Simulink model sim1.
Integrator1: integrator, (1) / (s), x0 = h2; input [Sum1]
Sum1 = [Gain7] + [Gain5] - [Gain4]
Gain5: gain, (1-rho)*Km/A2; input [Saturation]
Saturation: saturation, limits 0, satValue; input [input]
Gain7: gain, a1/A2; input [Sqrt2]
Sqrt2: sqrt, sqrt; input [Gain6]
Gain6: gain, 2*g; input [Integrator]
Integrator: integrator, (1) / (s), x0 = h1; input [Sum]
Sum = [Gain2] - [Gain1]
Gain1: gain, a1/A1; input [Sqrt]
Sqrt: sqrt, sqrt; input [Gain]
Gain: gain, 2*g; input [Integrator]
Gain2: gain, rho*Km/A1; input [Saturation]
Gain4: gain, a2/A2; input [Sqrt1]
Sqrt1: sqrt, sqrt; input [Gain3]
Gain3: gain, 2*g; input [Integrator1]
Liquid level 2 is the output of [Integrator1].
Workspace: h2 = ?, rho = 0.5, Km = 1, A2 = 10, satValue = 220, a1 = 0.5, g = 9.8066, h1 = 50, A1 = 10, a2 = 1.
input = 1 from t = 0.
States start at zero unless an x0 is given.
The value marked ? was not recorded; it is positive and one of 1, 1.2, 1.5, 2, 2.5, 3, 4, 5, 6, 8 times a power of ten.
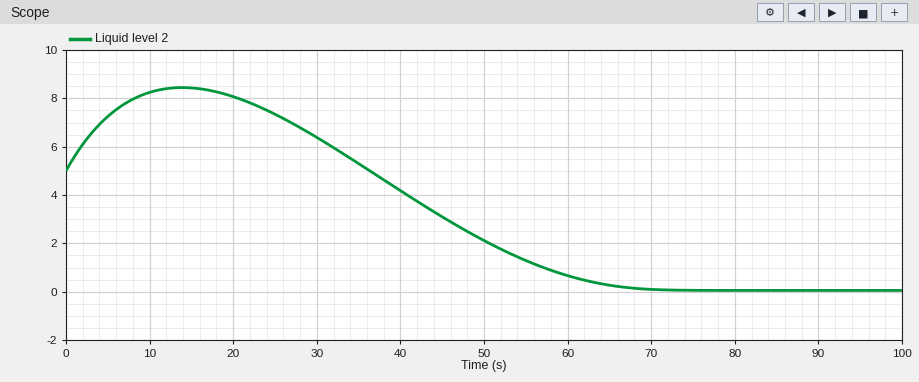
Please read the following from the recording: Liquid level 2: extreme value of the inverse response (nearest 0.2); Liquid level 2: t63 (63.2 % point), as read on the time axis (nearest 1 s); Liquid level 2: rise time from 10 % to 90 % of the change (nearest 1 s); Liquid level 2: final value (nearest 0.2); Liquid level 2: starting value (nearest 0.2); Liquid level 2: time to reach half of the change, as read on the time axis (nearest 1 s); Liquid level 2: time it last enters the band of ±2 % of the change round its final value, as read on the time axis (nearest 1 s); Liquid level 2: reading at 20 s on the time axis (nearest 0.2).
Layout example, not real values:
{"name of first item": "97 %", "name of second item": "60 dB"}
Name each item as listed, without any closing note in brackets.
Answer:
{"Liquid level 2: extreme value of the inverse response": "8.4", "Liquid level 2: t63 (63.2 % point), as read on the time axis": "51 s", "Liquid level 2: rise time from 10 % to 90 % of the change": "23 s", "Liquid level 2: final value": "0.0", "Liquid level 2: starting value": "5.0", "Liquid level 2: time to reach half of the change, as read on the time axis": "48 s", "Liquid level 2: time it last enters the band of ±2 % of the change round its final value, as read on the time axis": "68 s", "Liquid level 2: reading at 20 s on the time axis": "8.0"}
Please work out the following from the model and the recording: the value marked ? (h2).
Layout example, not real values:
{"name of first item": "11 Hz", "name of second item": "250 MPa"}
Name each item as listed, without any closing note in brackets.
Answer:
{"the value marked ?": "5"}
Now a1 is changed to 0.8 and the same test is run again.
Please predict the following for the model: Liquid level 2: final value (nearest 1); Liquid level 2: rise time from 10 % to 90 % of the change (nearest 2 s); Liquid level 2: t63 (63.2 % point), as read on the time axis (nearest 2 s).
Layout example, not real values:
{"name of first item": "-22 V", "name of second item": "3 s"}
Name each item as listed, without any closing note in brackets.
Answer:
{"Liquid level 2: final value": "0", "Liquid level 2: rise time from 10 % to 90 % of the change": "8 s", "Liquid level 2: t63 (63.2 % point), as read on the time axis": "42 s"}
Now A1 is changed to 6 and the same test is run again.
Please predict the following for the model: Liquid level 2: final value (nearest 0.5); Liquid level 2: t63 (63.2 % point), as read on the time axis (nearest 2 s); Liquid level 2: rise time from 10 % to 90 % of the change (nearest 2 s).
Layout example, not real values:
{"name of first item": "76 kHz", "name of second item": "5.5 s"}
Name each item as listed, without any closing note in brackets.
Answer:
{"Liquid level 2: final value": "0.0", "Liquid level 2: t63 (63.2 % point), as read on the time axis": "34 s", "Liquid level 2: rise time from 10 % to 90 % of the change": "14 s"}
